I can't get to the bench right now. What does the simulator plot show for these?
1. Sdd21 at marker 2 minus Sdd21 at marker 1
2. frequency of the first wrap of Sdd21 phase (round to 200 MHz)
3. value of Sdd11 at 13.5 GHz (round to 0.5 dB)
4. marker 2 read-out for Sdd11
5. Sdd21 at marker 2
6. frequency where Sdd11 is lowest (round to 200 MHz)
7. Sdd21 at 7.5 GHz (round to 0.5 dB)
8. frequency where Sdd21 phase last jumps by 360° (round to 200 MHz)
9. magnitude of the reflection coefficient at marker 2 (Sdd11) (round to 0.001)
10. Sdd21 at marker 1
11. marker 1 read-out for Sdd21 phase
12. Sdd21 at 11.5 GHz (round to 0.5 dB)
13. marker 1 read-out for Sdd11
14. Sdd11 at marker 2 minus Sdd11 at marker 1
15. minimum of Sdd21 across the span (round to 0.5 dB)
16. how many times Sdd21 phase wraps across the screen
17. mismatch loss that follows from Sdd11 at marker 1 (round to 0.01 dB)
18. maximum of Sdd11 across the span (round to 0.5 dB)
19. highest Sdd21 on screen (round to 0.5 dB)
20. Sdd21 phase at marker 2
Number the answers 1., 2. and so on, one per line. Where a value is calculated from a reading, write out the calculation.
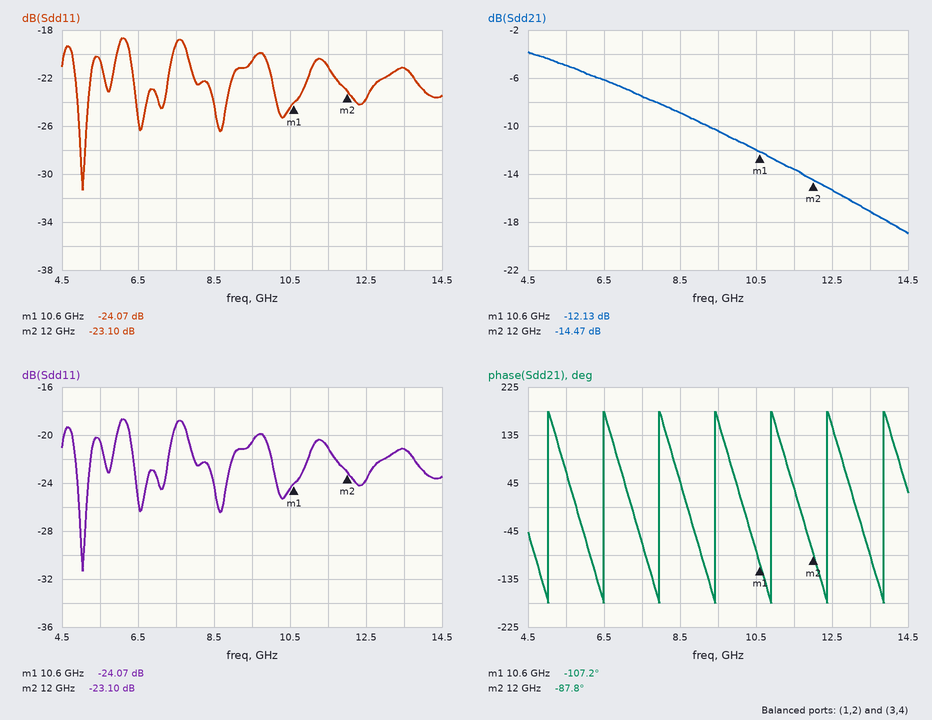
1. -14.47 − (-12.13) = -2.34 dB
2. 5.0 GHz
3. -21.0 dB
4. -23.10 dB
5. -14.47 dB
6. 5.0 GHz
7. -7.5 dB
8. 13.8 GHz
9. 10^(-23.1/20) ≈ 0.070
10. -12.13 dB
11. -107.2°
12. -13.5 dB
13. -24.07 dB
14. -23.1 − (-24.07) = 0.97 dB
15. -19.0 dB
16. 7
17. −10 log10(1 − 10^(-24.07/10)) ≈ 0.02 dB
18. -18.5 dB
19. -4.0 dB
20. -87.8°
